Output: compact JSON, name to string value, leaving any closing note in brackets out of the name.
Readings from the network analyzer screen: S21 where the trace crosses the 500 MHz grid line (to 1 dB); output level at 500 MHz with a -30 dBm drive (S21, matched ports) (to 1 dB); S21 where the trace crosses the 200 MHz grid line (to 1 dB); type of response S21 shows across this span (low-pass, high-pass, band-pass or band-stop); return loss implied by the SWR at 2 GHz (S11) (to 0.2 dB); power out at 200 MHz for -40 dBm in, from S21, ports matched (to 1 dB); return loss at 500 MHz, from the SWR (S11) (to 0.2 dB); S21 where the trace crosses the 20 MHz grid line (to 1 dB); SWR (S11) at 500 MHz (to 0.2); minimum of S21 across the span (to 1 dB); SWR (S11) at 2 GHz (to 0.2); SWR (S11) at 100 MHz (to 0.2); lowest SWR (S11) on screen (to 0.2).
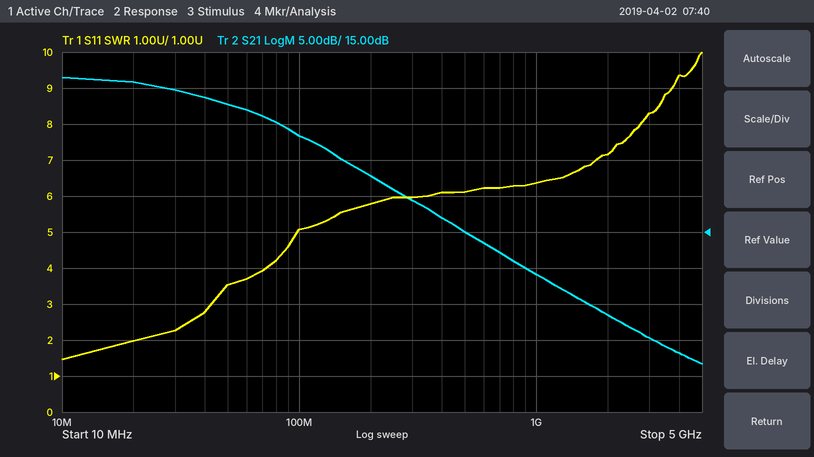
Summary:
{"S21 where the trace crosses the 500 MHz grid line": "15 dB", "output level at 500 MHz with a -30 dBm drive (S21, matched ports)": "-15 dBm", "S21 where the trace crosses the 200 MHz grid line": "23 dB", "type of response S21 shows across this span": "low-pass", "return loss implied by the SWR at 2 GHz (S11)": "2.4 dB", "power out at 200 MHz for -40 dBm in, from S21, ports matched": "-17 dBm", "return loss at 500 MHz, from the SWR (S11)": "2.8 dB", "S21 where the trace crosses the 20 MHz grid line": "36 dB", "SWR (S11) at 500 MHz": "6.2", "minimum of S21 across the span": "-3 dB", "SWR (S11) at 2 GHz": "7.2", "SWR (S11) at 100 MHz": "5.0", "lowest SWR (S11) on screen": "1.4"}
